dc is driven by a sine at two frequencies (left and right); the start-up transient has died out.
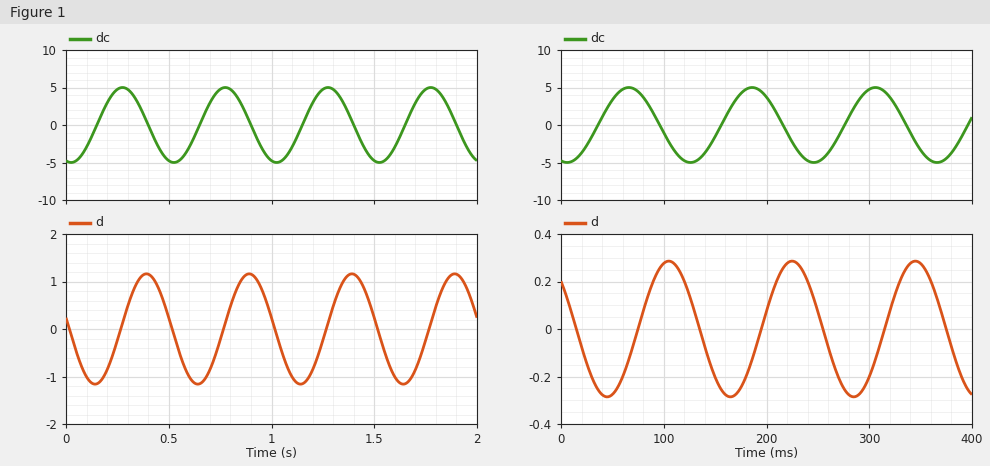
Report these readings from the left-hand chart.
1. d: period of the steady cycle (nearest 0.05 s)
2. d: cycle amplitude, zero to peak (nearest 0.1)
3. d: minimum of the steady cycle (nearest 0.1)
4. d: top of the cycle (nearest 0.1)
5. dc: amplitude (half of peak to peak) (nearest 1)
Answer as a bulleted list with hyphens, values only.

- 0.50 s
- 1.2
- -1.2
- 1.2
- 5
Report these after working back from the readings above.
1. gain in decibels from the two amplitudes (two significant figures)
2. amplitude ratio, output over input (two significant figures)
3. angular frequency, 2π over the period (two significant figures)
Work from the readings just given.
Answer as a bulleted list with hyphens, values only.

- -12 dB
- 0.24
- 13 rad/s
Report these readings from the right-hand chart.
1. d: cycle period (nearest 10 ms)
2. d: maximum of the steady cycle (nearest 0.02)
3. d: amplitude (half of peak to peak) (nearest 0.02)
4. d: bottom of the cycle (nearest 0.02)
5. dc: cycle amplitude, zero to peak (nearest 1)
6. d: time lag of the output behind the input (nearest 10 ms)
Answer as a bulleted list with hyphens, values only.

- 120 ms
- 0.28
- 0.28
- -0.28
- 5
- 40 ms
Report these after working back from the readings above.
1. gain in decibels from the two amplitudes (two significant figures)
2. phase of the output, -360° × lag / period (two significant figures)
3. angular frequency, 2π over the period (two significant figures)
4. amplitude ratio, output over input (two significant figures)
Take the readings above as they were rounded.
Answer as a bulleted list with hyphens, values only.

- -25 dB
- -120°
- 0.052 rad/ms
- 0.056
